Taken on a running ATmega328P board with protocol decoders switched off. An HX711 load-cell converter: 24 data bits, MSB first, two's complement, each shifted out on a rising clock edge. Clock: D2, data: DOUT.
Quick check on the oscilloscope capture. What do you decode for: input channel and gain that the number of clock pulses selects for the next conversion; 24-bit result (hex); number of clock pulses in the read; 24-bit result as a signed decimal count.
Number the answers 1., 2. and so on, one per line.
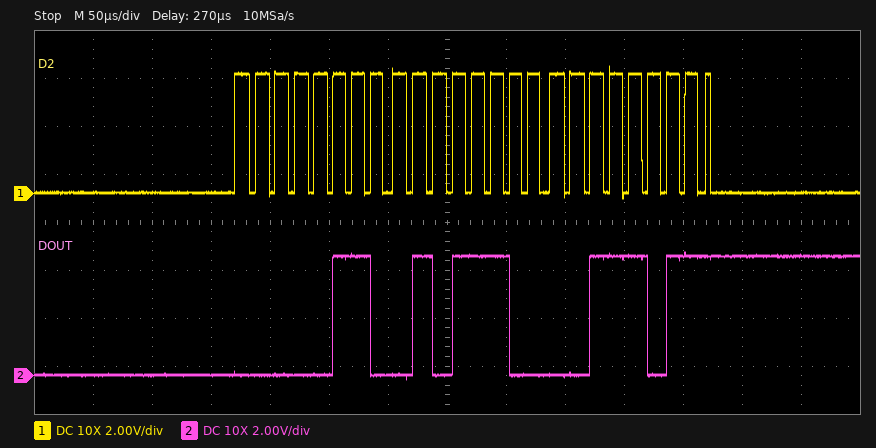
1. channel A, gain 128
2. 0x065C3B
3. 25
4. 416827
